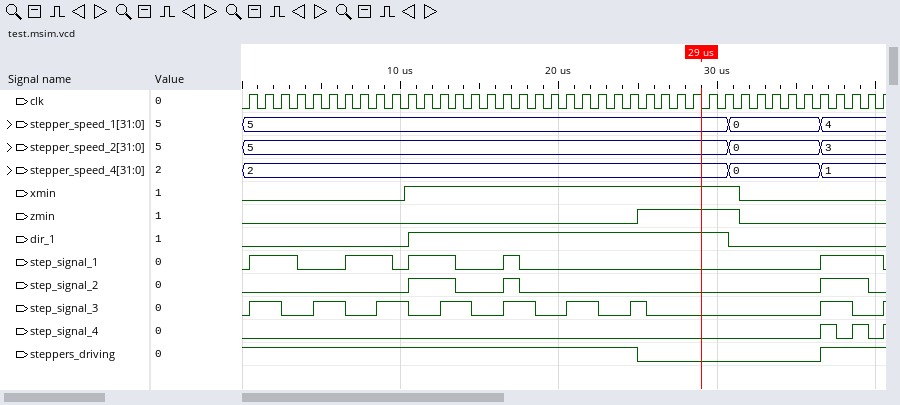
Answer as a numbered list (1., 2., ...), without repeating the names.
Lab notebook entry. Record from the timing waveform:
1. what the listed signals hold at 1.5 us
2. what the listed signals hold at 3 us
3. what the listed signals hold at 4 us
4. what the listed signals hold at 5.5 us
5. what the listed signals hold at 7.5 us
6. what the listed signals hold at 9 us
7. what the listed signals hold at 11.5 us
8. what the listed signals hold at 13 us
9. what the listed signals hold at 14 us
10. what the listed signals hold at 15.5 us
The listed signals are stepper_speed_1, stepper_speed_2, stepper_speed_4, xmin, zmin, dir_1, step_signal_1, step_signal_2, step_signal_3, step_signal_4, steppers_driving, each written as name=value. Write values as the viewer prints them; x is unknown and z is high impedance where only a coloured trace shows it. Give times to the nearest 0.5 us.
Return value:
1. stepper_speed_1=5, stepper_speed_2=5, stepper_speed_4=2, xmin=0, zmin=0, dir_1=0, step_signal_1=1, step_signal_2=0, step_signal_3=1, step_signal_4=0, steppers_driving=1
2. stepper_speed_1=5, stepper_speed_2=5, stepper_speed_4=2, xmin=0, zmin=0, dir_1=0, step_signal_1=1, step_signal_2=0, step_signal_3=0, step_signal_4=0, steppers_driving=1
3. stepper_speed_1=5, stepper_speed_2=5, stepper_speed_4=2, xmin=0, zmin=0, dir_1=0, step_signal_1=0, step_signal_2=0, step_signal_3=0, step_signal_4=0, steppers_driving=1
4. stepper_speed_1=5, stepper_speed_2=5, stepper_speed_4=2, xmin=0, zmin=0, dir_1=0, step_signal_1=0, step_signal_2=0, step_signal_3=1, step_signal_4=0, steppers_driving=1
5. stepper_speed_1=5, stepper_speed_2=5, stepper_speed_4=2, xmin=0, zmin=0, dir_1=0, step_signal_1=1, step_signal_2=0, step_signal_3=0, step_signal_4=0, steppers_driving=1
6. stepper_speed_1=5, stepper_speed_2=5, stepper_speed_4=2, xmin=0, zmin=0, dir_1=0, step_signal_1=1, step_signal_2=0, step_signal_3=1, step_signal_4=0, steppers_driving=1
7. stepper_speed_1=5, stepper_speed_2=5, stepper_speed_4=2, xmin=1, zmin=0, dir_1=1, step_signal_1=1, step_signal_2=1, step_signal_3=0, step_signal_4=0, steppers_driving=1
8. stepper_speed_1=5, stepper_speed_2=5, stepper_speed_4=2, xmin=1, zmin=0, dir_1=1, step_signal_1=1, step_signal_2=1, step_signal_3=1, step_signal_4=0, steppers_driving=1
9. stepper_speed_1=5, stepper_speed_2=5, stepper_speed_4=2, xmin=1, zmin=0, dir_1=1, step_signal_1=0, step_signal_2=0, step_signal_3=1, step_signal_4=0, steppers_driving=1
10. stepper_speed_1=5, stepper_speed_2=5, stepper_speed_4=2, xmin=1, zmin=0, dir_1=1, step_signal_1=0, step_signal_2=0, step_signal_3=0, step_signal_4=0, steppers_driving=1
